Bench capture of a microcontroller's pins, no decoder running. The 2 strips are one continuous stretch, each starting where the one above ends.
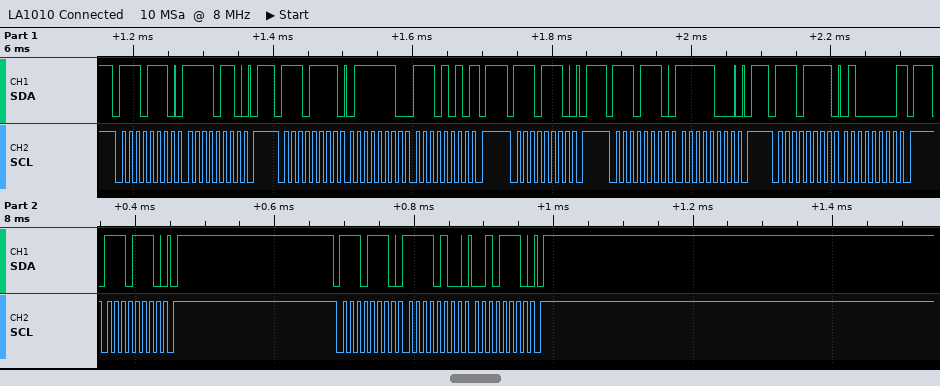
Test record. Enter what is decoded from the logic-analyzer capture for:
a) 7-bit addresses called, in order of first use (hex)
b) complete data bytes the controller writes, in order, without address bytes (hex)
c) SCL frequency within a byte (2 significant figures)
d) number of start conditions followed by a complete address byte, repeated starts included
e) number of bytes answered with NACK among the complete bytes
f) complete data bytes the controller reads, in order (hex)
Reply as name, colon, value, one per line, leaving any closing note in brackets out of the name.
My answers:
7-bit addresses called, in order of first use: 0x77
complete data bytes the controller writes, in order, without address bytes: F6 F8 F4 2E
SCL frequency within a byte: 100 kHz
number of start conditions followed by a complete address byte, repeated starts included: 7
number of bytes answered with NACK among the complete bytes: 2
complete data bytes the controller reads, in order: 7E EA 40
